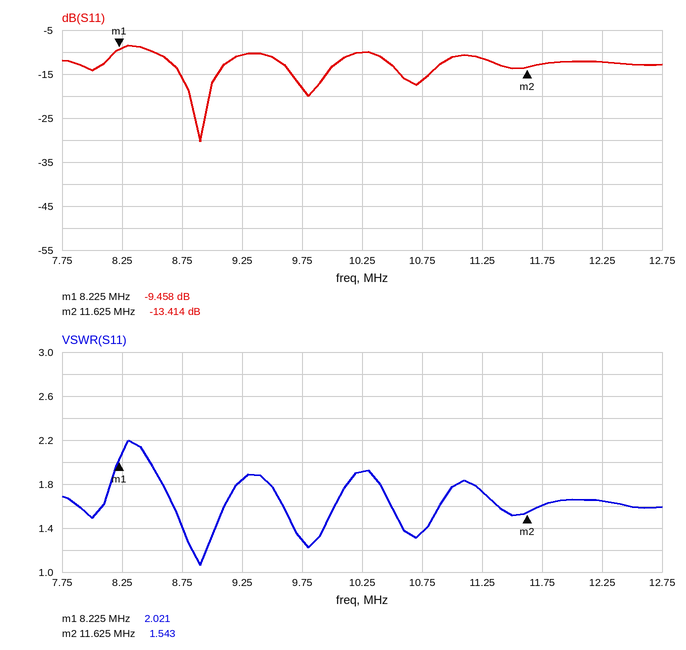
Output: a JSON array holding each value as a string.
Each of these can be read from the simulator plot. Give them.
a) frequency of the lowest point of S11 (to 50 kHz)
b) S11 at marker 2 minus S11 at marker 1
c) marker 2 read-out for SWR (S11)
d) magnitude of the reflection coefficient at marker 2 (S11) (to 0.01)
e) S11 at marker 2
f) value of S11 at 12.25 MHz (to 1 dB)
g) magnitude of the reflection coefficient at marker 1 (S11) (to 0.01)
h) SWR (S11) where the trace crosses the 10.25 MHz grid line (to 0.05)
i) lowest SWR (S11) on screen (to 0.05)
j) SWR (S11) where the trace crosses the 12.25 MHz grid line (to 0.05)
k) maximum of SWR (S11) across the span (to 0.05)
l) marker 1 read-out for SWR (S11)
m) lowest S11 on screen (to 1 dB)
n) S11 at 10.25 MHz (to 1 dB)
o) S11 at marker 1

["8.90 MHz", "-3.956 dB", "1.543", "0.21", "-13.414 dB", "-12 dB", "0.34", "1.90", "1.05", "1.65", "2.20", "2.021", "-30 dB", "-10 dB", "-9.458 dB"]
